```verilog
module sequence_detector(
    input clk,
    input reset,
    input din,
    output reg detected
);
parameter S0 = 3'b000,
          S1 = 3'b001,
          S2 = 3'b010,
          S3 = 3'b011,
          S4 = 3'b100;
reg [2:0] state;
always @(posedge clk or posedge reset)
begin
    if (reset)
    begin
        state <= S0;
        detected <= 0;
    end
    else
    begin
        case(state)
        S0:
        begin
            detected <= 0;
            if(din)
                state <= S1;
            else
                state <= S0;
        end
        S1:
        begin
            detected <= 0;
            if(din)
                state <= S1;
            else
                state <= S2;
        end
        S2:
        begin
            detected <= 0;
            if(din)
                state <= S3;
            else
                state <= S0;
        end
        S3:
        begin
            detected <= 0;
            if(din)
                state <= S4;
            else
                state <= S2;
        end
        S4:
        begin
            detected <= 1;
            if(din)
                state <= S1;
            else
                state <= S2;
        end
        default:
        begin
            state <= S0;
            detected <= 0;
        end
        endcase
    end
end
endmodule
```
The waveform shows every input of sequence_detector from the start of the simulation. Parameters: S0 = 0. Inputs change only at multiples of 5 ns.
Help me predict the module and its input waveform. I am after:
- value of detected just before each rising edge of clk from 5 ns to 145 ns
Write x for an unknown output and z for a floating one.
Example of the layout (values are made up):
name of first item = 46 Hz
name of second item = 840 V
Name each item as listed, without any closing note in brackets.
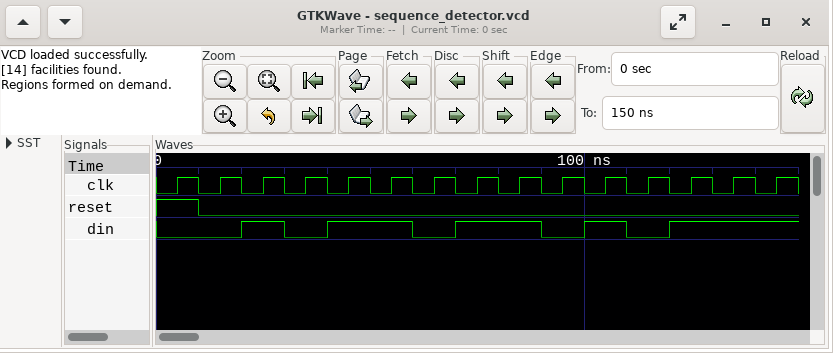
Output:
value of detected just before each rising edge of clk from 5 ns to 145 ns = 0 0 0 0 0 0 0 1 0 0 1 0 0 0 0
